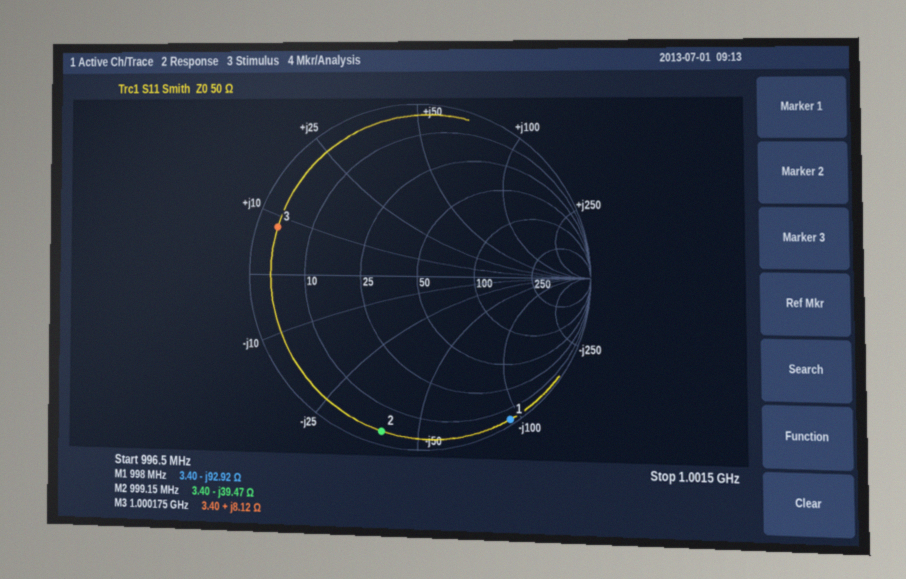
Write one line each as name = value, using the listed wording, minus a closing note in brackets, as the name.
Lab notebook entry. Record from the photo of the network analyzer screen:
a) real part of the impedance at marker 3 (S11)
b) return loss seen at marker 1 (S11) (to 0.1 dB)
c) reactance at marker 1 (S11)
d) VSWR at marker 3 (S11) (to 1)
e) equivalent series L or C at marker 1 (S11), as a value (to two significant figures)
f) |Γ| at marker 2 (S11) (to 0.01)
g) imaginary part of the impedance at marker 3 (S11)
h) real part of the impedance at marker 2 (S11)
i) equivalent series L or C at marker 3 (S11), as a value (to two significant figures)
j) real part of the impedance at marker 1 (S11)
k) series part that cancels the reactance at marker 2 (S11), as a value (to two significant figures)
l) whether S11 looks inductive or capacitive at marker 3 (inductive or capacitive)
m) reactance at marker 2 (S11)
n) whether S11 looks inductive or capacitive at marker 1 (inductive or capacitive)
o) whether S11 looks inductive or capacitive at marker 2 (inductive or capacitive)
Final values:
real part of the impedance at marker 3 = 3.40 Ω
return loss seen at marker 1 (S11) = 0.3 dB
reactance at marker 1 = -92.92 Ω
VSWR at marker 3 (S11) = 15
equivalent series L or C at marker 1 (S11), as a value = 1.7 pF
|Γ| at marker 2 (S11) = 0.92
imaginary part of the impedance at marker 3 = +8.12 Ω
real part of the impedance at marker 2 = 3.40 Ω
equivalent series L or C at marker 3 (S11), as a value = 1.3 nH
real part of the impedance at marker 1 = 3.40 Ω
series part that cancels the reactance at marker 2 (S11), as a value = 6.3 nH
whether S11 looks inductive or capacitive at marker 3 = inductive
reactance at marker 2 = -39.47 Ω
whether S11 looks inductive or capacitive at marker 1 = capacitive
whether S11 looks inductive or capacitive at marker 2 = capacitive
